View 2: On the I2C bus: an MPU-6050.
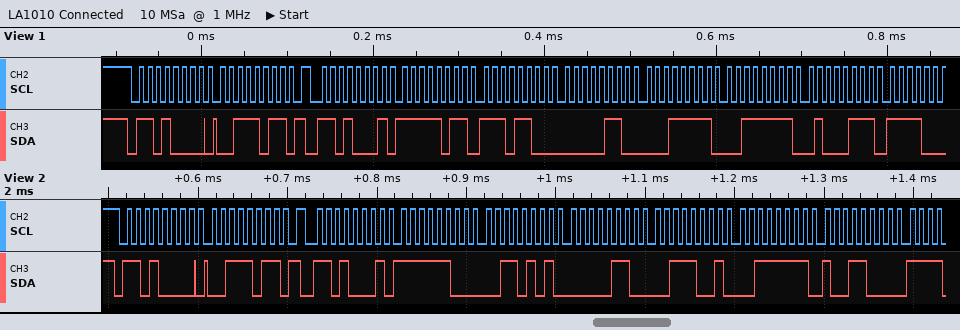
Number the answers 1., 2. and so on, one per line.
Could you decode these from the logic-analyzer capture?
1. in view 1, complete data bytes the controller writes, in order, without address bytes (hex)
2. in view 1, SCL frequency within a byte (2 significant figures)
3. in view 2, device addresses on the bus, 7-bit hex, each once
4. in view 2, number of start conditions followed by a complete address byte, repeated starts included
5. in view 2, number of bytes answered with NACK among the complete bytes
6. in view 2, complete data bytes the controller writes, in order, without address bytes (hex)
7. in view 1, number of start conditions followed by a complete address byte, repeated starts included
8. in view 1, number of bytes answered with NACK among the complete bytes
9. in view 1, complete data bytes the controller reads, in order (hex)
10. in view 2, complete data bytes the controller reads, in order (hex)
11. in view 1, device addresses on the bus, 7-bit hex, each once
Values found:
1. 3B
2. 100 kHz
3. 0x68
4. 2
5. 0
6. 3B
7. 2
8. 0
9. FB EC 06 1F 3F 47
10. FC 35 06 39 3F 98
11. 0x68
